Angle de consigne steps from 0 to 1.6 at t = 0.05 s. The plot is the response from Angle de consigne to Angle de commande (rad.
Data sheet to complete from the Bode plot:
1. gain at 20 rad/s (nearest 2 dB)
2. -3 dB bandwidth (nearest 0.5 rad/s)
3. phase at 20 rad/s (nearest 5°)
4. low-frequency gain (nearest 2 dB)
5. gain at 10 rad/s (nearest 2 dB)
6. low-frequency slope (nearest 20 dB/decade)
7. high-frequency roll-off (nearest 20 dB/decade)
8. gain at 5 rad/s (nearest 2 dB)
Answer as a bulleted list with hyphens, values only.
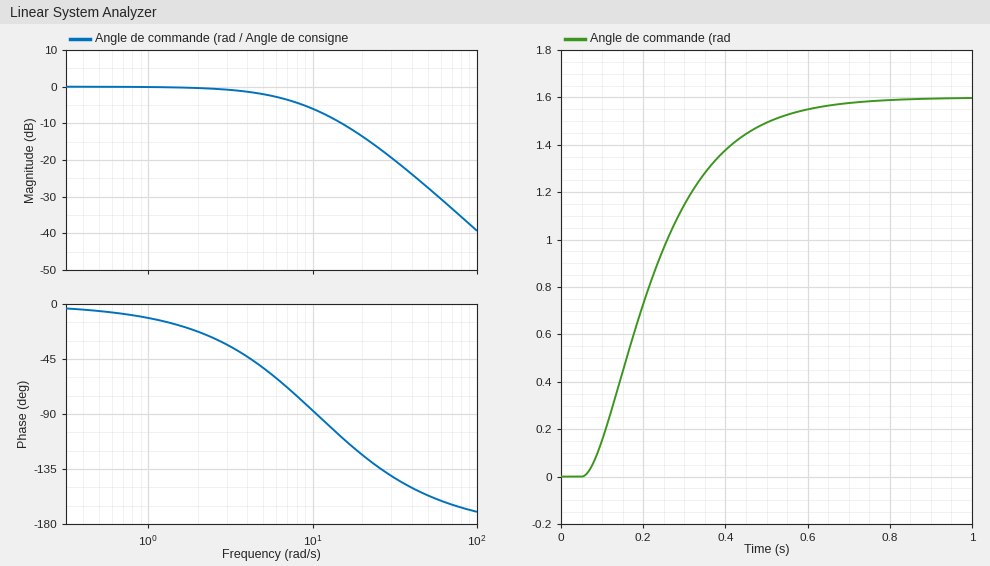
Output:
- -14 dB
- 6.5 rad/s
- -125°
- 0 dB
- -6 dB
- 0 dB/decade
- -40 dB/decade
- -2 dB
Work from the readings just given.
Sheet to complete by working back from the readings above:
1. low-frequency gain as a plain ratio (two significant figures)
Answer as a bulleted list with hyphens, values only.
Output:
- 1.0
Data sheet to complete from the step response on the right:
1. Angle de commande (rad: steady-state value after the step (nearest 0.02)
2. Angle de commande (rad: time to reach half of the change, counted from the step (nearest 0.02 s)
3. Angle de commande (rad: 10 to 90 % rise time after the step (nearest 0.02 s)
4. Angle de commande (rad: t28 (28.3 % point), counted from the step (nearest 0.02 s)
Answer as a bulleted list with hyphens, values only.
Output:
- 1.60
- 0.16 s
- 0.34 s
- 0.10 s
